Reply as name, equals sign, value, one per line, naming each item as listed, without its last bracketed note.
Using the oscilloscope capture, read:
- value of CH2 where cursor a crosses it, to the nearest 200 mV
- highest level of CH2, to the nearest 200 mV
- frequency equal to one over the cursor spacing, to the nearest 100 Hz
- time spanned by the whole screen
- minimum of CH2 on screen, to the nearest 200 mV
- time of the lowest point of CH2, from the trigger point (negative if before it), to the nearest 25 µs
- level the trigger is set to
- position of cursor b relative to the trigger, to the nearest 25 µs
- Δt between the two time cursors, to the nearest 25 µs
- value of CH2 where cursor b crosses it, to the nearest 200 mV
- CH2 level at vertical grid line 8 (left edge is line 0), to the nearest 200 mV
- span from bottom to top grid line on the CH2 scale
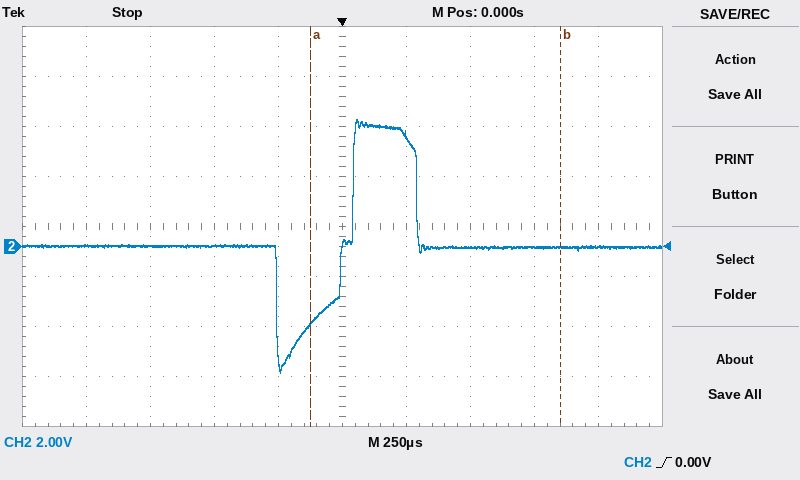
value of CH2 where cursor a crosses it, to the nearest 200 mV = -3.0 V
highest level of CH2, to the nearest 200 mV = 5.0 V
frequency equal to one over the cursor spacing, to the nearest 100 Hz = 1.0 kHz
time spanned by the whole screen = 2.5 ms
minimum of CH2 on screen, to the nearest 200 mV = -5.0 V
time of the lowest point of CH2, from the trigger point (negative if before it), to the nearest 25 µs = -250 µs
level the trigger is set to = 0.00 V
position of cursor b relative to the trigger, to the nearest 25 µs = +850 µs
Δt between the two time cursors, to the nearest 25 µs = 975 µs
value of CH2 where cursor b crosses it, to the nearest 200 mV = 0.0 V
CH2 level at vertical grid line 8 (left edge is line 0), to the nearest 200 mV = 0.0 V
span from bottom to top grid line on the CH2 scale = 16 V
